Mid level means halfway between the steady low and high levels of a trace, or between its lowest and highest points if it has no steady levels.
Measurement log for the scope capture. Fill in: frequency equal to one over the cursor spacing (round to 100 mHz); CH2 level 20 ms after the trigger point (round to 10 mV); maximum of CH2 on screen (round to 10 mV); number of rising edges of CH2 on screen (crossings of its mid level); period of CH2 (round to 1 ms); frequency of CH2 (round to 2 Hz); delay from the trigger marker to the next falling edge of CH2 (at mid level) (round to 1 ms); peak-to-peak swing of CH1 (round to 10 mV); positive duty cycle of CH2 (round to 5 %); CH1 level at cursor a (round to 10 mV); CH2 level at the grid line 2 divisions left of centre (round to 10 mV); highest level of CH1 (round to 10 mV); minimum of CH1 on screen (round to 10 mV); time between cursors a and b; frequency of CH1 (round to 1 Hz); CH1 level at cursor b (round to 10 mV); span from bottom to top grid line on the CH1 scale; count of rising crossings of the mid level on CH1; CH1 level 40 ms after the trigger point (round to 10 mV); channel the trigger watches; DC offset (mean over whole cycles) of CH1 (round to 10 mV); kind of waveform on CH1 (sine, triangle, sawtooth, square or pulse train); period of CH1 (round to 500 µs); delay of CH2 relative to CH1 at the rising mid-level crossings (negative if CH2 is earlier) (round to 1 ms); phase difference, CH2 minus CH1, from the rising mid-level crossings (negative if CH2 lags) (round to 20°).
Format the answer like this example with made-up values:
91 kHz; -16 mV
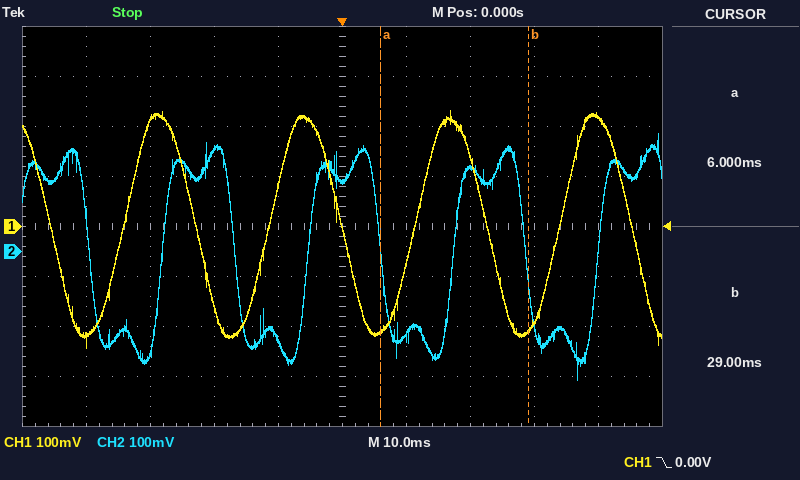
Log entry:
43.5 Hz; 170 mV; 240 mV; 4; 23 ms; 44 Hz; 6 ms; 470 mV; 50 %; -210 mV; 200 mV; 230 mV; -240 mV; 23 ms; 44 Hz; -210 mV; 800 mV; 4; 220 mV; CH1; 0 mV; sine; 22.5 ms; +6 ms; -100°
